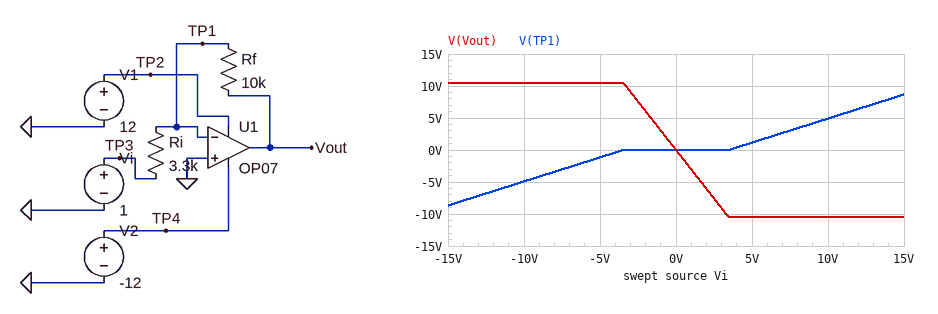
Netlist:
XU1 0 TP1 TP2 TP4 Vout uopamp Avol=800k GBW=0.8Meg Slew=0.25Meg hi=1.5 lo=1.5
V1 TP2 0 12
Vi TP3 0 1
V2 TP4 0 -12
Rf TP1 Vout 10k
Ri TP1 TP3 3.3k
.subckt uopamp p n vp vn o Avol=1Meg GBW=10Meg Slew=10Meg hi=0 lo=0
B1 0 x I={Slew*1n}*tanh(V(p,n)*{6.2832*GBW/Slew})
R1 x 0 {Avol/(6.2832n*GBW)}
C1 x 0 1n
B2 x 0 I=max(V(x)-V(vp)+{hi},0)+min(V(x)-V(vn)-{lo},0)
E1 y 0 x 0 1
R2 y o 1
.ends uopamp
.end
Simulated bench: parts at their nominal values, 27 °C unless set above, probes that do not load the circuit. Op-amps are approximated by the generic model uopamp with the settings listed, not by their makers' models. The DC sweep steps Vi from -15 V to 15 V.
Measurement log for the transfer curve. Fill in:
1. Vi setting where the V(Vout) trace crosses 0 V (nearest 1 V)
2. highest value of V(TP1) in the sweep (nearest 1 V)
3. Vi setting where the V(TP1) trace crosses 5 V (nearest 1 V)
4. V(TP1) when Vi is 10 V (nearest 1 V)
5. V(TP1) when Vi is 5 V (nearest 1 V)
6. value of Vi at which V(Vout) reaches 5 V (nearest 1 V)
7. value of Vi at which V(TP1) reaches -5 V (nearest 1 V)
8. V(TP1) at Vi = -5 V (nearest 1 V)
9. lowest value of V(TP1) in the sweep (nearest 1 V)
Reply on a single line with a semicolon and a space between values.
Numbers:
0 V; 9 V; 10 V; 5 V; 1 V; -2 V; -10 V; -1 V; -9 V
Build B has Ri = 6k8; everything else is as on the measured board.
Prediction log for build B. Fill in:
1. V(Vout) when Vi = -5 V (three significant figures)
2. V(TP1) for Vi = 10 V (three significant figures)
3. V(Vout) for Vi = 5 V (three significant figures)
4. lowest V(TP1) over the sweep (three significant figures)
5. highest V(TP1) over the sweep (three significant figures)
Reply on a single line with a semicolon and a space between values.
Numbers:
7.35 V; 1.70 V; -7.35 V; -4.68 V; 4.68 V
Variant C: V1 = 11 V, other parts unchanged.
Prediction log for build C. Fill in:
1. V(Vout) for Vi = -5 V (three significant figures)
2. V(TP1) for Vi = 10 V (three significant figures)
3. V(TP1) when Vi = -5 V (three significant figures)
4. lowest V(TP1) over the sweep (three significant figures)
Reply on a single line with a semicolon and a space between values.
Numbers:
9.50 V; 4.91 V; -1.40 V; -8.92 V
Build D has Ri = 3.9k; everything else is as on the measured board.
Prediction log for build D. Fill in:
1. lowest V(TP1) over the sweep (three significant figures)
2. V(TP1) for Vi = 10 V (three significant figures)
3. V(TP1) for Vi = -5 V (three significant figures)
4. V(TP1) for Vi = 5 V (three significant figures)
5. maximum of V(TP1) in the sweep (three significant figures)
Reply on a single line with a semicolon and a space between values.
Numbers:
-7.85 V; 4.25 V; -651 mV; 651 mV; 7.85 V
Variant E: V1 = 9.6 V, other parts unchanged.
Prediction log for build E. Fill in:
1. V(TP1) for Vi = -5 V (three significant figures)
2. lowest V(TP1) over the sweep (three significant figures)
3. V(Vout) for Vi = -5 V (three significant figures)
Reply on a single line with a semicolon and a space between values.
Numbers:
-1.75 V; -9.27 V; 8.10 V
